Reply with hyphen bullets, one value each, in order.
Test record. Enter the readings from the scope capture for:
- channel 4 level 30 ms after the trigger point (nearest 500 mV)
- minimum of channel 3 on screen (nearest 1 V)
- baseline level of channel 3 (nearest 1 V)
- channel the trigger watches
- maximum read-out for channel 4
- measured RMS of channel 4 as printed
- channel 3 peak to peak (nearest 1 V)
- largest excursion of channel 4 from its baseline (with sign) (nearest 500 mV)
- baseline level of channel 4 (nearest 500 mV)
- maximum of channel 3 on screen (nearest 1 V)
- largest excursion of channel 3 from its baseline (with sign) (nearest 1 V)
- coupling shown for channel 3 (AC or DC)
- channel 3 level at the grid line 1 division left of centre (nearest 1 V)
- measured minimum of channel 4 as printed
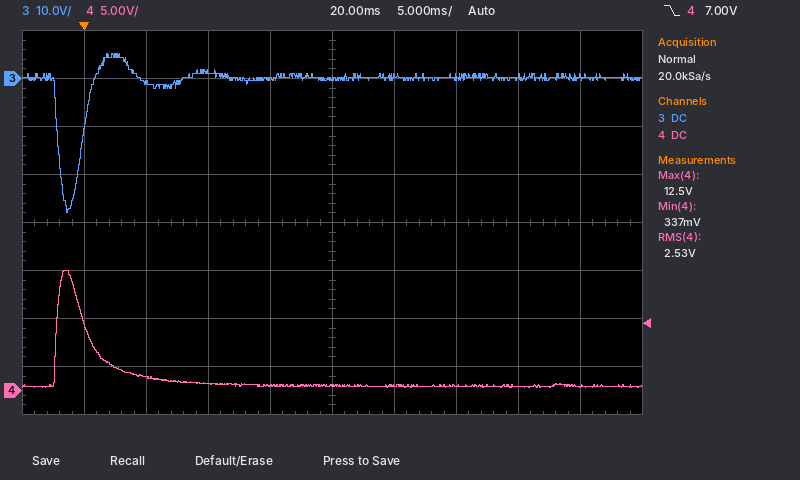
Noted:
- 500 mV
- -28 V
- 0 V
- channel 4
- 12.5 V
- 2.53 V
- 33 V
- +12.0 V
- 500 mV
- 5 V
- -28 V
- DC
- 0 V
- 337 mV
